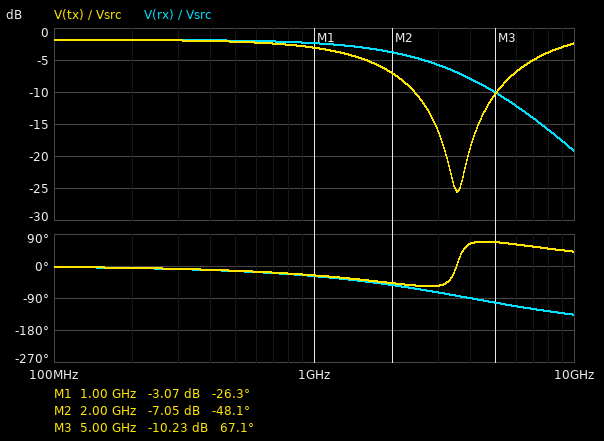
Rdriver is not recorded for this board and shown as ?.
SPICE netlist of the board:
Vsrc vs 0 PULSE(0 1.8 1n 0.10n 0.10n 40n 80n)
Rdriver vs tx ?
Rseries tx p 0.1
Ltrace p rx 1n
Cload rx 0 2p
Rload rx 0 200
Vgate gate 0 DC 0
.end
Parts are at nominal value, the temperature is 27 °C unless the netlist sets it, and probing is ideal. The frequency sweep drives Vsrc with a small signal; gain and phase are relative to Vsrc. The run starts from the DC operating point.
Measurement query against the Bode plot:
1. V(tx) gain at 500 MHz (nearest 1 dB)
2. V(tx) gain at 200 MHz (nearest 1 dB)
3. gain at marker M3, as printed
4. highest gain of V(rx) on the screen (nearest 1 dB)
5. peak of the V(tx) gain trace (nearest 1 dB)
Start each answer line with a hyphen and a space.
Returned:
- -2 dB
- -2 dB
- -10.23 dB
- -2 dB
- -2 dB
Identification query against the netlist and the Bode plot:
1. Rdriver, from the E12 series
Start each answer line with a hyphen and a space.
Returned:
- 47 Ω
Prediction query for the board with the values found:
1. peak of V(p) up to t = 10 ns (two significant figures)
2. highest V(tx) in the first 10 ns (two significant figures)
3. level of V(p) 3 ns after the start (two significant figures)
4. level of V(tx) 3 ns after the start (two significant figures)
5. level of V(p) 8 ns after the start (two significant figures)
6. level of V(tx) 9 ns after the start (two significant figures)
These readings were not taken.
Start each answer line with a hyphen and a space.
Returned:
- 1.5 V
- 1.5 V
- 1.5 V
- 1.5 V
- 1.5 V
- 1.5 V
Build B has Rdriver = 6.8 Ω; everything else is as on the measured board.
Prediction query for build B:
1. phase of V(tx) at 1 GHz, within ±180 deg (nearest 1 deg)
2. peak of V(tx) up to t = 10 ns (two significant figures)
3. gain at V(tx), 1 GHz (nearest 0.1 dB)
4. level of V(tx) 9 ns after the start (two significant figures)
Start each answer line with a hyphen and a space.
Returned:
- -5 deg
- 1.9 V
- -0.4 dB
- 1.7 V
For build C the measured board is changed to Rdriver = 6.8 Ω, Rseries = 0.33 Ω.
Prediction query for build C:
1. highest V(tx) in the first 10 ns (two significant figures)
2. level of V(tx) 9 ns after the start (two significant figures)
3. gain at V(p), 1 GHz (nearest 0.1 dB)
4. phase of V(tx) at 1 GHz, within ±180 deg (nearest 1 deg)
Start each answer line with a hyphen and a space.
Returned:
- 1.9 V
- 1.7 V
- -0.4 dB
- -5 deg
